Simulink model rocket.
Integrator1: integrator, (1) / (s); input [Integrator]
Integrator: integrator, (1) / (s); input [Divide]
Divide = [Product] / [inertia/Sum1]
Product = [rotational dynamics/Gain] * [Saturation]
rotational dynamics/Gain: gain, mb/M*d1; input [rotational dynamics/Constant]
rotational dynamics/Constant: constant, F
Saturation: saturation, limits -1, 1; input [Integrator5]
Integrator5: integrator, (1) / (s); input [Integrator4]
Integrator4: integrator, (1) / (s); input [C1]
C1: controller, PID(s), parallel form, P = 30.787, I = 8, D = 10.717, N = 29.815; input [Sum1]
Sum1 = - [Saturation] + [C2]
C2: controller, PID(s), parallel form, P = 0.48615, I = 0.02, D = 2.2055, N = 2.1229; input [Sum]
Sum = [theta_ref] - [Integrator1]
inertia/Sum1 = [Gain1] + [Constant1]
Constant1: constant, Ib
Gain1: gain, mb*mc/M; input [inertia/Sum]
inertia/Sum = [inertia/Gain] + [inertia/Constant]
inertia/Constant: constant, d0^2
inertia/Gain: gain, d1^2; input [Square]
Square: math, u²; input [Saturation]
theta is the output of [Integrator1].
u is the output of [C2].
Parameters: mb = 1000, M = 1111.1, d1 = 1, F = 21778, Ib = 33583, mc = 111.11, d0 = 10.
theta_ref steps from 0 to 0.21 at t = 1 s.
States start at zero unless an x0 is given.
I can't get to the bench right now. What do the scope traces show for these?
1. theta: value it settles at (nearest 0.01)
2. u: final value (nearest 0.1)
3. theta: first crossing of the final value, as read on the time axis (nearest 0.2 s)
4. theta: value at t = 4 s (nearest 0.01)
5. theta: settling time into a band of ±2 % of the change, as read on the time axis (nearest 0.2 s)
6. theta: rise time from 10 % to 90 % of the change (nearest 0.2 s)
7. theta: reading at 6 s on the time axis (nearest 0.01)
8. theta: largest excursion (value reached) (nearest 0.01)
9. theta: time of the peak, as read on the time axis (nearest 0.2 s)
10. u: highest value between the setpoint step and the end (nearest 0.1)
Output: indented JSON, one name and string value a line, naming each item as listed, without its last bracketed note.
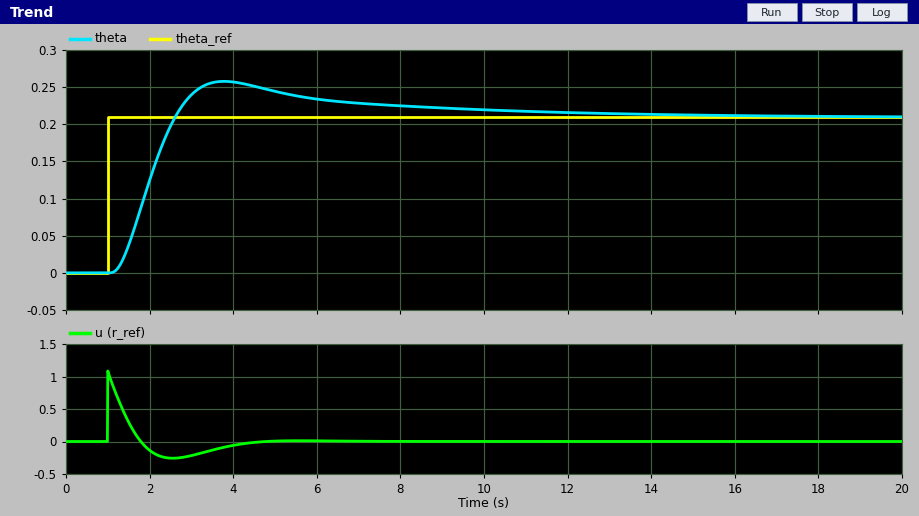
{
  "theta: value it settles at": "0.21",
  "u: final value": "0.0",
  "theta: first crossing of the final value, as read on the time axis": "2.6 s",
  "theta: value at t = 4 s": "0.26",
  "theta: settling time into a band of ±2 % of the change, as read on the time axis": "13.2 s",
  "theta: rise time from 10 % to 90 % of the change": "1.0 s",
  "theta: reading at 6 s on the time axis": "0.23",
  "theta: largest excursion (value reached)": "0.26",
  "theta: time of the peak, as read on the time axis": "3.8 s",
  "u: highest value between the setpoint step and the end": "1.1"
}
